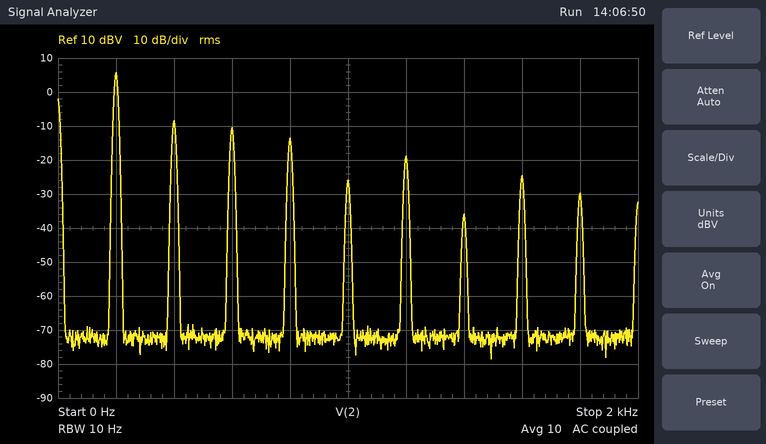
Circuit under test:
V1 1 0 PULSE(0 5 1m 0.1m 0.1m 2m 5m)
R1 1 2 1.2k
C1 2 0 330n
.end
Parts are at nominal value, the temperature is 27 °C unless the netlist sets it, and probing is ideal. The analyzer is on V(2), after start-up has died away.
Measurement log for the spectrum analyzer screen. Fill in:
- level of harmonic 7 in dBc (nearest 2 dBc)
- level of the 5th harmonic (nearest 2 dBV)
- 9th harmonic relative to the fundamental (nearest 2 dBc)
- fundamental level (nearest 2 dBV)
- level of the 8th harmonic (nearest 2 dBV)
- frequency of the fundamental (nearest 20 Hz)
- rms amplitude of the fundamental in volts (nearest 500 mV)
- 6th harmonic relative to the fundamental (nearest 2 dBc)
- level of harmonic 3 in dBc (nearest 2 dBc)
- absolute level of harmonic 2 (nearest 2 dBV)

-42 dBc
-26 dBV
-36 dBc
6 dBV
-24 dBV
200 Hz
2.0 V
-24 dBc
-16 dBc
-8 dBV
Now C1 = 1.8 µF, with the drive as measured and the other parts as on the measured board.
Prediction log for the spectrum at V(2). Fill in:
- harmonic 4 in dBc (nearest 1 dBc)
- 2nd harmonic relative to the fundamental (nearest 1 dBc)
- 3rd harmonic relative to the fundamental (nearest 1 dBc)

-25 dBc
-18 dBc
-21 dBc
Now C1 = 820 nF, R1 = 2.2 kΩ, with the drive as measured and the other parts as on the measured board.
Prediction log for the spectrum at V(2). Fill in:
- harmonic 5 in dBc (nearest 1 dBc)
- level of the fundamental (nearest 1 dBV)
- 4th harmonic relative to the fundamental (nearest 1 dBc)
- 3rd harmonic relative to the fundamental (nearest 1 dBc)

-37 dBc
-1 dBV
-25 dBc
-21 dBc
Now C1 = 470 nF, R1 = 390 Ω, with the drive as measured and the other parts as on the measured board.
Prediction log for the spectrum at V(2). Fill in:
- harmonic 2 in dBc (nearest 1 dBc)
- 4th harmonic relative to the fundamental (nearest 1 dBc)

-13 dBc
-16 dBc
